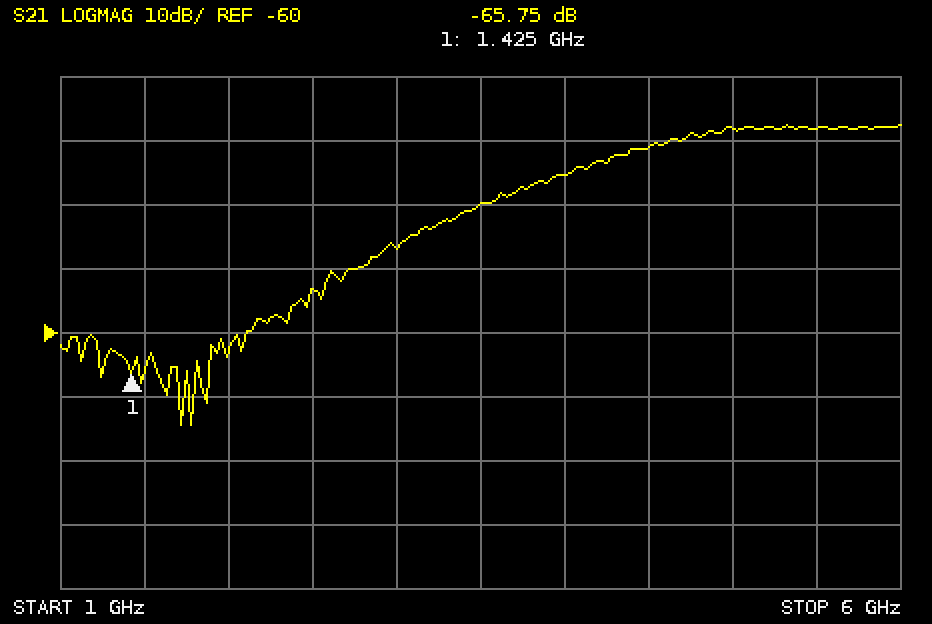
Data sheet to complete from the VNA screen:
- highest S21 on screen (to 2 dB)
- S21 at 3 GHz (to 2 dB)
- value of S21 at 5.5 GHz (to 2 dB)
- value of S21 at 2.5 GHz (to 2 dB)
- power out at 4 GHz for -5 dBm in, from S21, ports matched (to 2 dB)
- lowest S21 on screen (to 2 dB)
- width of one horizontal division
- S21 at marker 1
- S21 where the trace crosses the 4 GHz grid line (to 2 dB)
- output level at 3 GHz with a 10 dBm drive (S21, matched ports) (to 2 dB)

-28 dB
-46 dB
-28 dB
-54 dB
-40 dBm
-74 dB
500 MHz
-65.75 dB
-36 dB
-36 dBm
